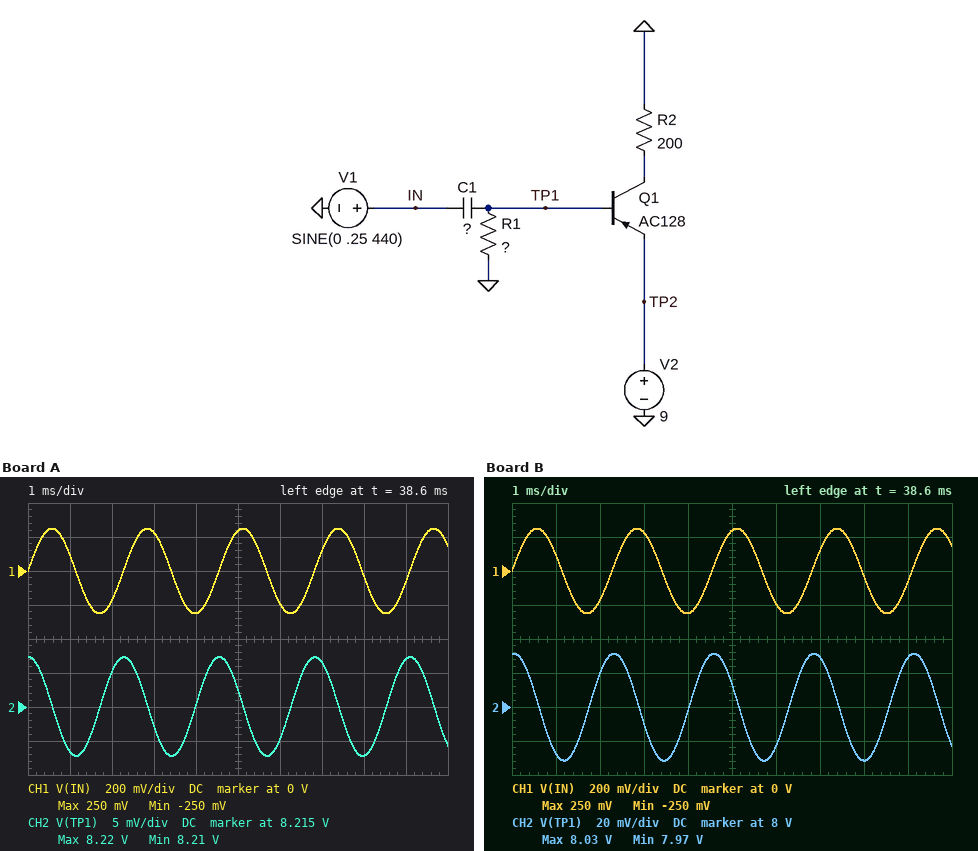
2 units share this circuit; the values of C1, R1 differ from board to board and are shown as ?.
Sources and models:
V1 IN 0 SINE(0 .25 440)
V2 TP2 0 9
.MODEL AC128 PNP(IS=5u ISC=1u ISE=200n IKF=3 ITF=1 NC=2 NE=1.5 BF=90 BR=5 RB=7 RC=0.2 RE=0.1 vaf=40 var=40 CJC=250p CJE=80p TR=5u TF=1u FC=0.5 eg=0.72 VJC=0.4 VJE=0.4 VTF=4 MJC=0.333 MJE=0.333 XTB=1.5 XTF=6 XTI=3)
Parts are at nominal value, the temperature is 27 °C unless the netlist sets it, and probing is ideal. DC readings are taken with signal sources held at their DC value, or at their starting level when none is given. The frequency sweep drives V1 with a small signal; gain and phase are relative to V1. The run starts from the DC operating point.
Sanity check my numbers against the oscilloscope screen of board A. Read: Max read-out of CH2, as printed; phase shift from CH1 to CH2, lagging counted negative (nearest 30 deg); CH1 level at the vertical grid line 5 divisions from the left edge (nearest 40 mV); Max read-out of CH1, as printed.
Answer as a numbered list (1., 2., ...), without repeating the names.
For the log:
1. 8.22 V
2. 90 deg
3. 240 mV
4. 250 mV
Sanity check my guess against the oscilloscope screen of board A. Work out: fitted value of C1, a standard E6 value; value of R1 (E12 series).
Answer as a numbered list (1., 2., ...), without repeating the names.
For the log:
1. 1.5 µF
2. 120 Ω
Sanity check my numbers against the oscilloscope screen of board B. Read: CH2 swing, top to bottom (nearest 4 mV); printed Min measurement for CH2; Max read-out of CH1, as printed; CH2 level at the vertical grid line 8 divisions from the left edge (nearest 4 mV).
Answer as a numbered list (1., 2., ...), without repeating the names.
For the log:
1. 64 mV
2. 7.97 V
3. 250 mV
4. 7.968 V
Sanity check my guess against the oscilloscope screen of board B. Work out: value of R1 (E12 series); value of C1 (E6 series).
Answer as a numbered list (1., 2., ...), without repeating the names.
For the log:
1. 82 Ω
2. 6.8 µF
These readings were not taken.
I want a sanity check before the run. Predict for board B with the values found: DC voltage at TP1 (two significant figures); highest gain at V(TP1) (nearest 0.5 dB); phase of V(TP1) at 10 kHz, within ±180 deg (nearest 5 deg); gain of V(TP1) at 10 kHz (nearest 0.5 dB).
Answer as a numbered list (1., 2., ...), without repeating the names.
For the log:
1. 8.0 V
2. 0 dB
3. 20 deg
4. -0.5 dB
